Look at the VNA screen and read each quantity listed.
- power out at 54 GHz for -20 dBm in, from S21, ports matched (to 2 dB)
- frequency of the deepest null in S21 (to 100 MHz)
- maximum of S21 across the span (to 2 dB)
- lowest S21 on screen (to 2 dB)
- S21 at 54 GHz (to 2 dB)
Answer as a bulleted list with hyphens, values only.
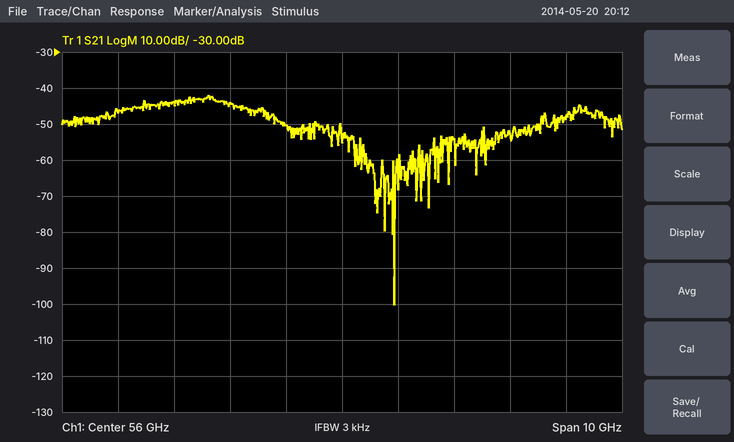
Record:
- -64 dBm
- 56.9 GHz
- -42 dB
- -100 dB
- -44 dB
